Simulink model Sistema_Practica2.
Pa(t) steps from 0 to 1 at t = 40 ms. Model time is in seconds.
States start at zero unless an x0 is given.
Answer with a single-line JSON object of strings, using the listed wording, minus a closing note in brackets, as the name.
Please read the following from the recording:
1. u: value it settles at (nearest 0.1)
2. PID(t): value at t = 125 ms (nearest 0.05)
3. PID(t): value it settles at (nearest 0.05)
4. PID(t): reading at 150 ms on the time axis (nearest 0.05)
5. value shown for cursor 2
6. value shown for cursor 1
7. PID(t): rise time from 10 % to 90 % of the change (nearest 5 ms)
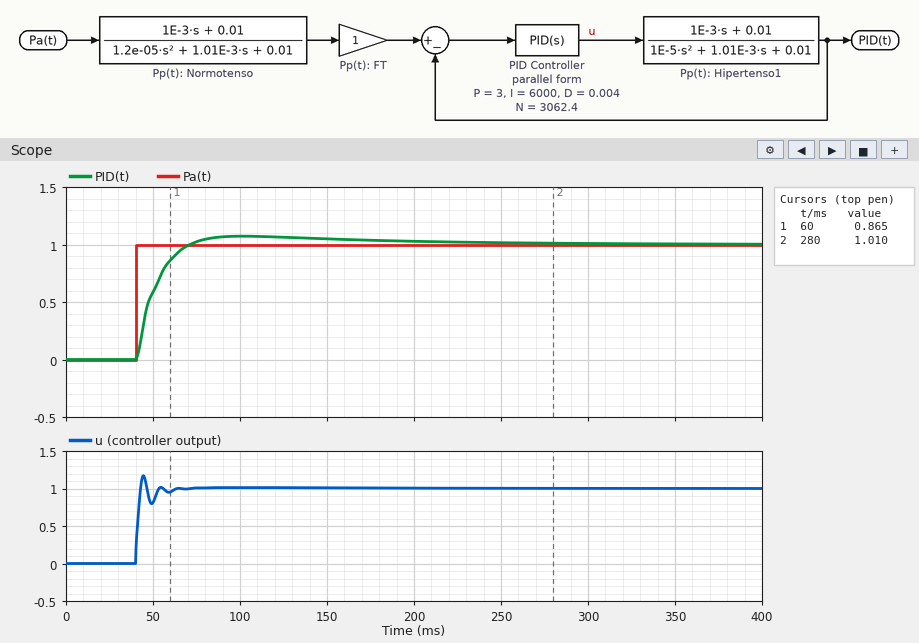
{"u: value it settles at": "1.0", "PID(t): value at t = 125 ms": "1.05", "PID(t): value it settles at": "1.00", "PID(t): reading at 150 ms on the time axis": "1.05", "value shown for cursor 2": "1.010", "value shown for cursor 1": "0.865", "PID(t): rise time from 10 % to 90 % of the change": "20 ms"}
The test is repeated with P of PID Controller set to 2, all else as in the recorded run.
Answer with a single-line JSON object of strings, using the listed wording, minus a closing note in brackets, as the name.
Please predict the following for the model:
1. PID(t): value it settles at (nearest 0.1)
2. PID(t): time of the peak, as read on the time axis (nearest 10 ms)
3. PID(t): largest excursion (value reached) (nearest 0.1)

{"PID(t): value it settles at": "1.0", "PID(t): time of the peak, as read on the time axis": "100 ms", "PID(t): largest excursion (value reached)": "1.1"}
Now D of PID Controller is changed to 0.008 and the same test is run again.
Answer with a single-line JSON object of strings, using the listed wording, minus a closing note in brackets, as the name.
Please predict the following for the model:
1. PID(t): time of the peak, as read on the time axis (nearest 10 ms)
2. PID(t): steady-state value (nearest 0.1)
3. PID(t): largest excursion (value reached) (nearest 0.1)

{"PID(t): time of the peak, as read on the time axis": "100 ms", "PID(t): steady-state value": "1.0", "PID(t): largest excursion (value reached)": "1.1"}
